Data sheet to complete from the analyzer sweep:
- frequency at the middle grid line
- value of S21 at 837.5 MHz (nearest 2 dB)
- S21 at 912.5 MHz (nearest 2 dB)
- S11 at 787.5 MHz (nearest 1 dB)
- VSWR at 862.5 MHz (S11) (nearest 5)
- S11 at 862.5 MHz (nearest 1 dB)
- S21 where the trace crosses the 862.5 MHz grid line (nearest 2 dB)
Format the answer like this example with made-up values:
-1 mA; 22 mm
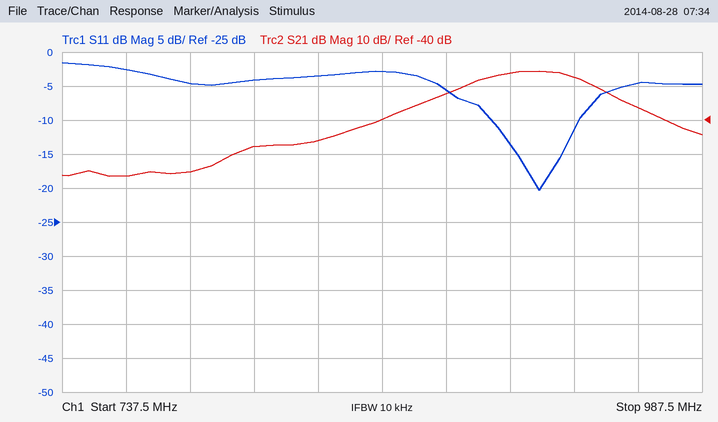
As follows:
862.5 MHz; -46 dB; -26 dB; -5 dB; 5; -3 dB; -40 dB
